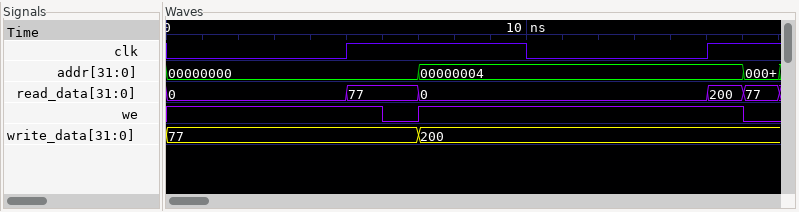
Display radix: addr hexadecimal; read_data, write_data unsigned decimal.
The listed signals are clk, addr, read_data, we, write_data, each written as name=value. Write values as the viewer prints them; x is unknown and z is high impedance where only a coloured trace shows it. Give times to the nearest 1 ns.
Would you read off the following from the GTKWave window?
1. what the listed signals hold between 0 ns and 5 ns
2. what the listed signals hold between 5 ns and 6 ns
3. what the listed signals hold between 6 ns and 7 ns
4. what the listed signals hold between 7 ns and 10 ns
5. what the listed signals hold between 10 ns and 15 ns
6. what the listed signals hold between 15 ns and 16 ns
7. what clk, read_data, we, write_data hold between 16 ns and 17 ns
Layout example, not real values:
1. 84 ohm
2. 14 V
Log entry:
1. clk=0, addr=00000000, read_data=0, we=1, write_data=77
2. clk=1, addr=00000000, read_data=77, we=1, write_data=77
3. clk=1, addr=00000000, read_data=77, we=0, write_data=77
4. clk=1, addr=00000004, read_data=0, we=1, write_data=200
5. clk=0, addr=00000004, read_data=0, we=1, write_data=200
6. clk=1, addr=00000004, read_data=200, we=1, write_data=200
7. clk=1, read_data=77, we=0, write_data=200
